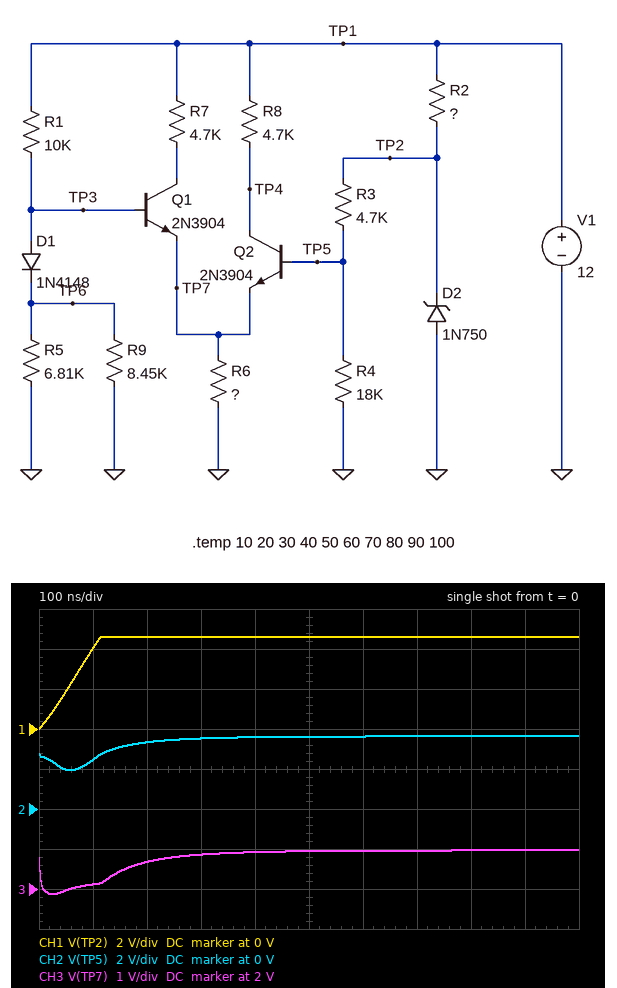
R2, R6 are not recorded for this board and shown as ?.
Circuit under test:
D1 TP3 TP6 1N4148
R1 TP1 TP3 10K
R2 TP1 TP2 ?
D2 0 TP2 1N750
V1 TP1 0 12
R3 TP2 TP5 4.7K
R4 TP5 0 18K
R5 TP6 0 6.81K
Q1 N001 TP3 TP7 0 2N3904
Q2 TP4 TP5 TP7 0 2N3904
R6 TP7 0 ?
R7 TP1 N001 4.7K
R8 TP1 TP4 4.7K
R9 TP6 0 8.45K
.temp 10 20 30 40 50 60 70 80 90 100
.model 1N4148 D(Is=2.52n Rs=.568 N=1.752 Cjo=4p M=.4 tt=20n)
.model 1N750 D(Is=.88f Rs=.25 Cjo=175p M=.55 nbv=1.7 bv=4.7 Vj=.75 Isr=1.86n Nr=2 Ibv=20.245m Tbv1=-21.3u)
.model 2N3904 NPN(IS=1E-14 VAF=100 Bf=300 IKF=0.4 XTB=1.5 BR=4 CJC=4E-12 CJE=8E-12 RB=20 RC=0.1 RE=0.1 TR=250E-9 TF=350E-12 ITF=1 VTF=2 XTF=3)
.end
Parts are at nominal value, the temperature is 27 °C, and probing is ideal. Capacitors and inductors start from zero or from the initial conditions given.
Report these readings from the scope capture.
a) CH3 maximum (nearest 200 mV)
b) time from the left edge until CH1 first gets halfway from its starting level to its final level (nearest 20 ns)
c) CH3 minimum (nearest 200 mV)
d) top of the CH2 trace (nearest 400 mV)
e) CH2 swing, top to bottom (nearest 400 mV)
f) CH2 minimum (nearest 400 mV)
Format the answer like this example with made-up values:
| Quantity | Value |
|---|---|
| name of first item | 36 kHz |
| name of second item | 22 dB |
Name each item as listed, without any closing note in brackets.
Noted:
| Quantity | Value |
|---|---|
| CH3 maximum | 3.0 V |
| time from the left edge until CH1 first gets halfway from its starting level to its final level | 60 ns |
| CH3 minimum | 1.8 V |
| top of the CH2 trace | 3.6 V |
| CH2 swing, top to bottom | 1.6 V |
| CH2 minimum | 2.0 V |
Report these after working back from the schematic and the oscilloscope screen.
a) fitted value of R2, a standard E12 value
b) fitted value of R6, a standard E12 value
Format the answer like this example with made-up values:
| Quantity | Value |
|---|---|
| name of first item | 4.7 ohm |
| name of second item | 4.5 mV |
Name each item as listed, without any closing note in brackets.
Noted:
| Quantity | Value |
|---|---|
| fitted value of R2, a standard E12 value | 2.7 kΩ |
| fitted value of R6, a standard E12 value | 820 Ω |
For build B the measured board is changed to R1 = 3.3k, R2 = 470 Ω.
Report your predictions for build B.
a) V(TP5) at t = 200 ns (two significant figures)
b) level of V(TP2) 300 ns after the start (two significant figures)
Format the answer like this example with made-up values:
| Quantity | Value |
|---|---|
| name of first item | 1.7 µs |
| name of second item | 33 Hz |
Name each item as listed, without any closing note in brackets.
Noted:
| Quantity | Value |
|---|---|
| V(TP5) at t = 200 ns | 3.7 V |
| level of V(TP2) 300 ns after the start | 4.7 V |
